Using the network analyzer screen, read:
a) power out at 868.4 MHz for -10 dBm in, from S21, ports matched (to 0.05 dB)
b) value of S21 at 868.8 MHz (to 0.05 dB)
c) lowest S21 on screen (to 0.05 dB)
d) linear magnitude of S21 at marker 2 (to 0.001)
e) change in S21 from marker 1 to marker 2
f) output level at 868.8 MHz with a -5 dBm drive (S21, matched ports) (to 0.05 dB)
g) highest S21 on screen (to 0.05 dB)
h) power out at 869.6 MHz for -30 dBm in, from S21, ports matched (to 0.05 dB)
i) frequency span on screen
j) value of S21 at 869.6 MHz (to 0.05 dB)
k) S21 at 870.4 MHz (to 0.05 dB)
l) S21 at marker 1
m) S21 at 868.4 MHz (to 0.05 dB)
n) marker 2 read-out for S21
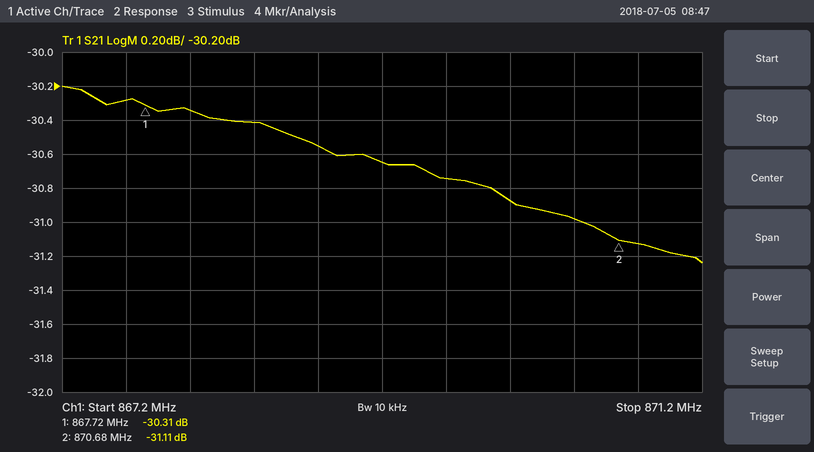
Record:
-40.40 dBm
-30.55 dB
-31.25 dB
0.028
-0.80 dB
-35.55 dBm
-30.20 dB
-60.75 dBm
4 MHz
-30.75 dB
-31.00 dB
-30.31 dB
-30.40 dB
-31.11 dB
